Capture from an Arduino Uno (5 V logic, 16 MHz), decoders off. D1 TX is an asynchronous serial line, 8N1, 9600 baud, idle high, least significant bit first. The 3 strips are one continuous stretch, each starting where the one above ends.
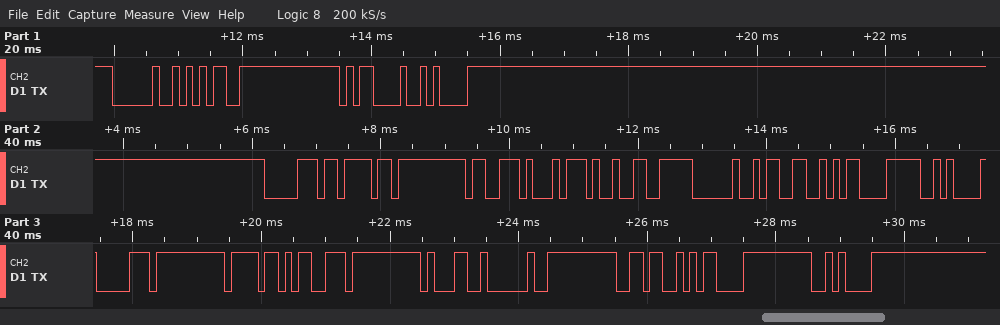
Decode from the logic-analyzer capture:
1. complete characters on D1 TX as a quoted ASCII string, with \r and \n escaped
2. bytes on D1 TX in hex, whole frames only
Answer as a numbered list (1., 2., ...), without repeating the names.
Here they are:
1. " 5\r\npost2 3\r\npos1 6\r\n"
2. 20 35 0D 0A 70 6F 73 74 32 20 33 0D 0A 70 6F 73 31 20 36 0D 0A
